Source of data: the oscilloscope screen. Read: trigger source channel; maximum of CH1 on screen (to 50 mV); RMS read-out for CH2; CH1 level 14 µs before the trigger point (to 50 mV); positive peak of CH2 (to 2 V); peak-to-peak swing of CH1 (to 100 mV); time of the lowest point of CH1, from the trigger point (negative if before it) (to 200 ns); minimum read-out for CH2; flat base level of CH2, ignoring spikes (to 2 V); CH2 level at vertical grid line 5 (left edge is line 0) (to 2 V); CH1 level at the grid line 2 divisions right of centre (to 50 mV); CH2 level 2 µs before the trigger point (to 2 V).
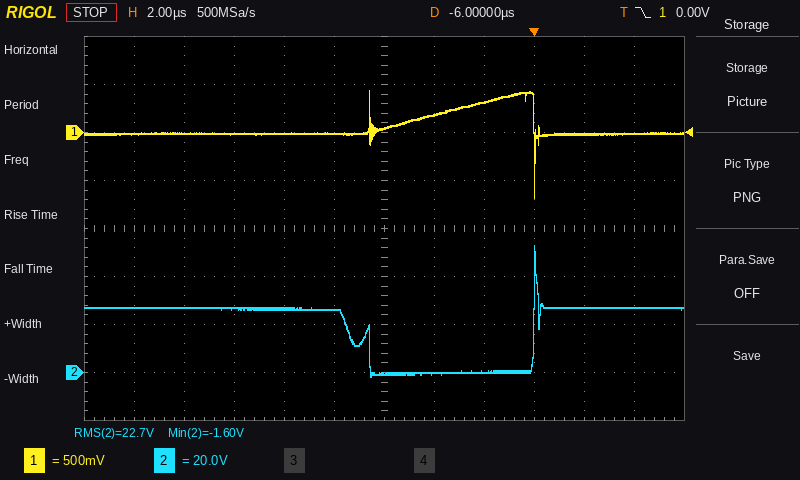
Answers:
CH1
450 mV
22.7 V
0 mV
52 V
1.10 V
0.0 µs
-1.60 V
0 V
26 V
300 mV
0 V
